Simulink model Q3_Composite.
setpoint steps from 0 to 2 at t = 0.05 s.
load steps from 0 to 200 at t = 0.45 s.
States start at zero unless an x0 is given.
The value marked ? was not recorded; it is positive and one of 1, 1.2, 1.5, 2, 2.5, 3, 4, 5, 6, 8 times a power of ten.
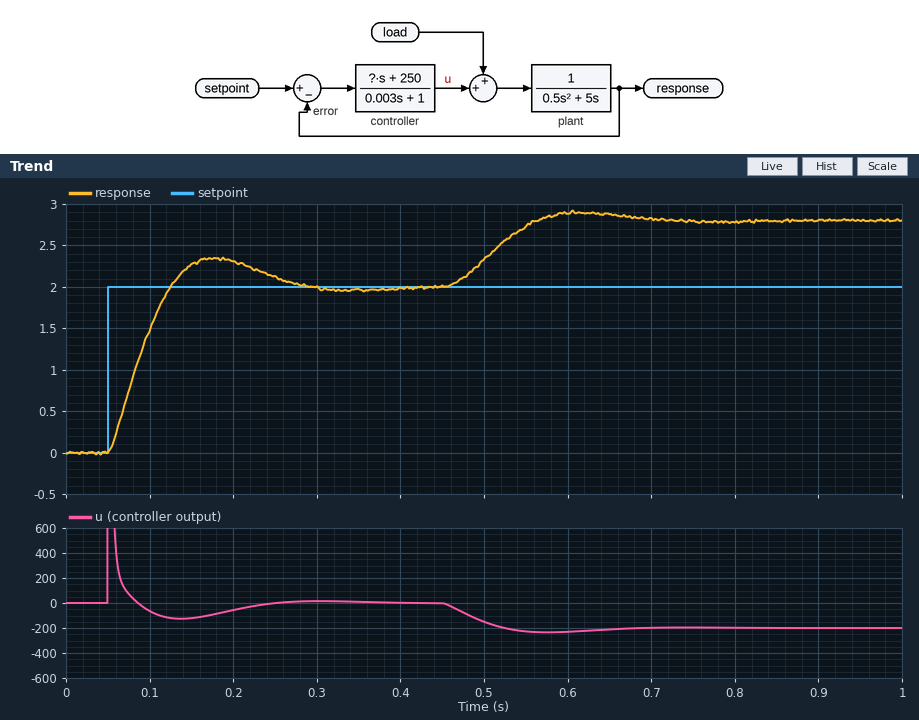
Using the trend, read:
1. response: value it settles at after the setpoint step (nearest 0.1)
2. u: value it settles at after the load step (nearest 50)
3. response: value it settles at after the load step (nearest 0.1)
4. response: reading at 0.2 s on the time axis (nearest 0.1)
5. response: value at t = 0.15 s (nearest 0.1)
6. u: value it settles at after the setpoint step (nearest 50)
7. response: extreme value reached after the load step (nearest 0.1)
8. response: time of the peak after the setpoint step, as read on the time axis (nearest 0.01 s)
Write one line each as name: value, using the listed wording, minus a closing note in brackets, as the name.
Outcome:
response: value it settles at after the setpoint step: 2.0
u: value it settles at after the load step: -200
response: value it settles at after the load step: 2.8
response: reading at 0.2 s on the time axis: 2.3
response: value at t = 0.15 s: 2.3
u: value it settles at after the setpoint step: 0
response: extreme value reached after the load step: 2.9
response: time of the peak after the setpoint step, as read on the time axis: 0.18 s
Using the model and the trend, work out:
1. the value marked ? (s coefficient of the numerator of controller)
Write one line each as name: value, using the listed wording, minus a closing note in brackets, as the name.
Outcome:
the value marked ?: 8
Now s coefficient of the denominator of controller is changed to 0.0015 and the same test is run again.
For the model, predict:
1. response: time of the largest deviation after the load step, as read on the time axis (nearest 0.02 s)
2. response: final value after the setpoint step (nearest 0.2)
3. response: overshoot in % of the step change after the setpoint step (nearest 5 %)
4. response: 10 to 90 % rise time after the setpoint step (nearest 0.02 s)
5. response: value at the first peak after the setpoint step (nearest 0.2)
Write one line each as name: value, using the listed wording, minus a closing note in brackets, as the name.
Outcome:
response: time of the largest deviation after the load step, as read on the time axis: 0.62 s
response: final value after the setpoint step: 2.0
response: overshoot in % of the step change after the setpoint step: 15 %
response: 10 to 90 % rise time after the setpoint step: 0.06 s
response: value at the first peak after the setpoint step: 2.4
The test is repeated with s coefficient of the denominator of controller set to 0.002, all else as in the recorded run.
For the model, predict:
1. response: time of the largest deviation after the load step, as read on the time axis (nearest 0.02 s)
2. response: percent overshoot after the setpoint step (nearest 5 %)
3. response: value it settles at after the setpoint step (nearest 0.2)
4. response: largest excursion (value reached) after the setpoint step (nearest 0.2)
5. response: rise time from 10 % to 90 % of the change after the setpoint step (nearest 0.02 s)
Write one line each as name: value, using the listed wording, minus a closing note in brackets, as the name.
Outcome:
response: time of the largest deviation after the load step, as read on the time axis: 0.62 s
response: percent overshoot after the setpoint step: 15 %
response: value it settles at after the setpoint step: 2.0
response: largest excursion (value reached) after the setpoint step: 2.4
response: rise time from 10 % to 90 % of the change after the setpoint step: 0.06 s
